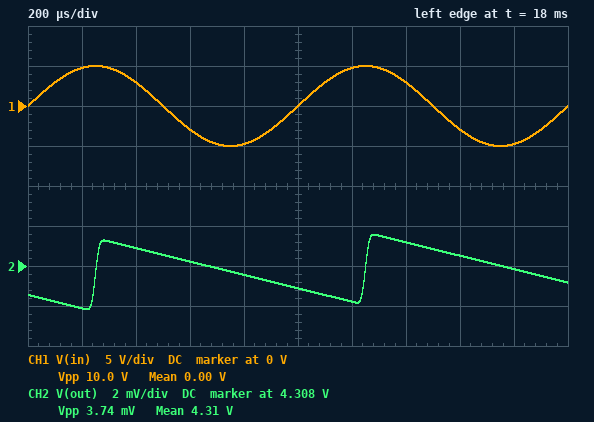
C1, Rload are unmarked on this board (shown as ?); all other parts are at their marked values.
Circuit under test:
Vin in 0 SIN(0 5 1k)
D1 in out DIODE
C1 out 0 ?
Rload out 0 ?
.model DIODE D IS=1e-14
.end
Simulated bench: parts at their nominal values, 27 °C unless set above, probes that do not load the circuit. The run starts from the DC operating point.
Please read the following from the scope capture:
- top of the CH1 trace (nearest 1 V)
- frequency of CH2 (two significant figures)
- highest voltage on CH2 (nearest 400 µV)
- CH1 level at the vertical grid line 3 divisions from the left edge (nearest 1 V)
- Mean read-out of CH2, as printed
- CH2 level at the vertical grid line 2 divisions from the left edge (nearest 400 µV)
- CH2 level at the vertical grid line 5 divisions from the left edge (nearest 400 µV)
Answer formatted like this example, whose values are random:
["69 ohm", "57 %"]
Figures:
["5 V", "1.0 kHz", "4.3096 V", "-3 V", "4.31 V", "4.3088 V", "4.3068 V"]
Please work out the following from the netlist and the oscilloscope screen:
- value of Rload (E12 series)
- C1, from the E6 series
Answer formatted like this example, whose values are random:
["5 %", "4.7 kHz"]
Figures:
["39 kΩ", "33 µF"]
